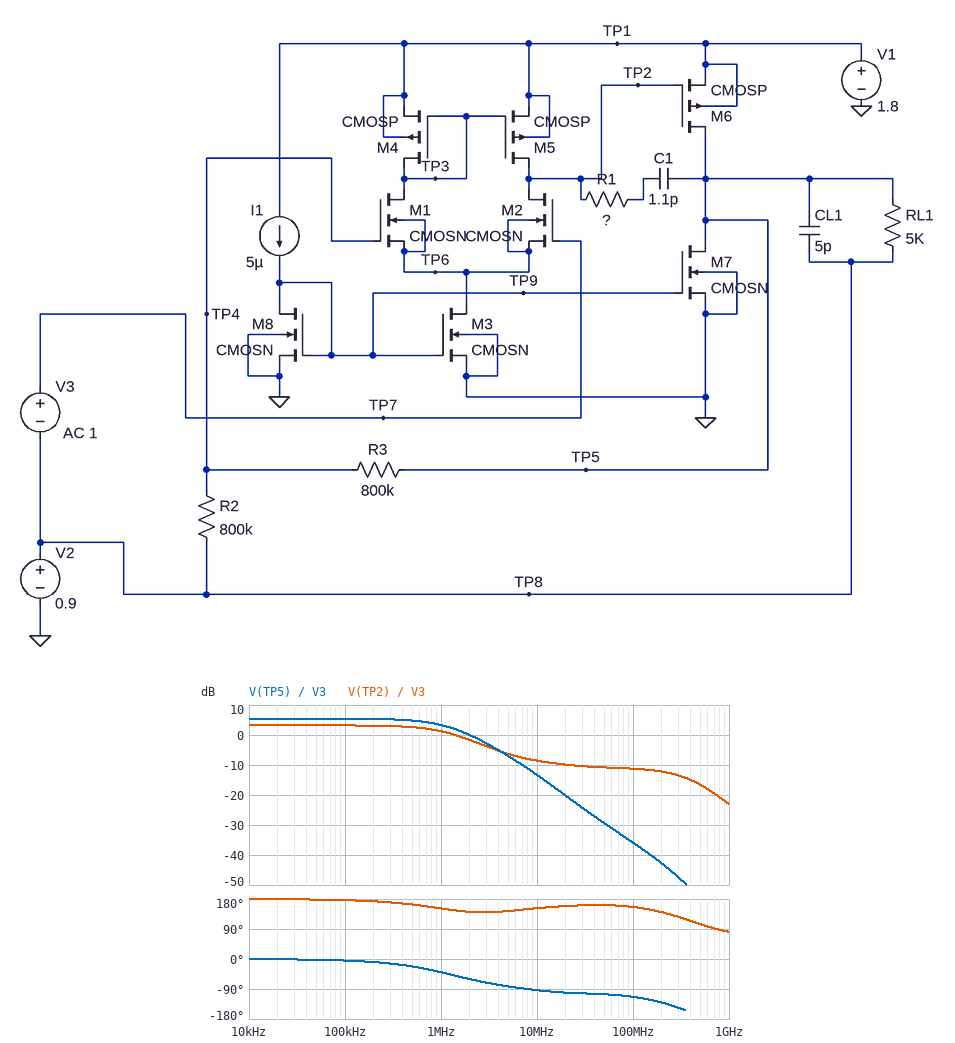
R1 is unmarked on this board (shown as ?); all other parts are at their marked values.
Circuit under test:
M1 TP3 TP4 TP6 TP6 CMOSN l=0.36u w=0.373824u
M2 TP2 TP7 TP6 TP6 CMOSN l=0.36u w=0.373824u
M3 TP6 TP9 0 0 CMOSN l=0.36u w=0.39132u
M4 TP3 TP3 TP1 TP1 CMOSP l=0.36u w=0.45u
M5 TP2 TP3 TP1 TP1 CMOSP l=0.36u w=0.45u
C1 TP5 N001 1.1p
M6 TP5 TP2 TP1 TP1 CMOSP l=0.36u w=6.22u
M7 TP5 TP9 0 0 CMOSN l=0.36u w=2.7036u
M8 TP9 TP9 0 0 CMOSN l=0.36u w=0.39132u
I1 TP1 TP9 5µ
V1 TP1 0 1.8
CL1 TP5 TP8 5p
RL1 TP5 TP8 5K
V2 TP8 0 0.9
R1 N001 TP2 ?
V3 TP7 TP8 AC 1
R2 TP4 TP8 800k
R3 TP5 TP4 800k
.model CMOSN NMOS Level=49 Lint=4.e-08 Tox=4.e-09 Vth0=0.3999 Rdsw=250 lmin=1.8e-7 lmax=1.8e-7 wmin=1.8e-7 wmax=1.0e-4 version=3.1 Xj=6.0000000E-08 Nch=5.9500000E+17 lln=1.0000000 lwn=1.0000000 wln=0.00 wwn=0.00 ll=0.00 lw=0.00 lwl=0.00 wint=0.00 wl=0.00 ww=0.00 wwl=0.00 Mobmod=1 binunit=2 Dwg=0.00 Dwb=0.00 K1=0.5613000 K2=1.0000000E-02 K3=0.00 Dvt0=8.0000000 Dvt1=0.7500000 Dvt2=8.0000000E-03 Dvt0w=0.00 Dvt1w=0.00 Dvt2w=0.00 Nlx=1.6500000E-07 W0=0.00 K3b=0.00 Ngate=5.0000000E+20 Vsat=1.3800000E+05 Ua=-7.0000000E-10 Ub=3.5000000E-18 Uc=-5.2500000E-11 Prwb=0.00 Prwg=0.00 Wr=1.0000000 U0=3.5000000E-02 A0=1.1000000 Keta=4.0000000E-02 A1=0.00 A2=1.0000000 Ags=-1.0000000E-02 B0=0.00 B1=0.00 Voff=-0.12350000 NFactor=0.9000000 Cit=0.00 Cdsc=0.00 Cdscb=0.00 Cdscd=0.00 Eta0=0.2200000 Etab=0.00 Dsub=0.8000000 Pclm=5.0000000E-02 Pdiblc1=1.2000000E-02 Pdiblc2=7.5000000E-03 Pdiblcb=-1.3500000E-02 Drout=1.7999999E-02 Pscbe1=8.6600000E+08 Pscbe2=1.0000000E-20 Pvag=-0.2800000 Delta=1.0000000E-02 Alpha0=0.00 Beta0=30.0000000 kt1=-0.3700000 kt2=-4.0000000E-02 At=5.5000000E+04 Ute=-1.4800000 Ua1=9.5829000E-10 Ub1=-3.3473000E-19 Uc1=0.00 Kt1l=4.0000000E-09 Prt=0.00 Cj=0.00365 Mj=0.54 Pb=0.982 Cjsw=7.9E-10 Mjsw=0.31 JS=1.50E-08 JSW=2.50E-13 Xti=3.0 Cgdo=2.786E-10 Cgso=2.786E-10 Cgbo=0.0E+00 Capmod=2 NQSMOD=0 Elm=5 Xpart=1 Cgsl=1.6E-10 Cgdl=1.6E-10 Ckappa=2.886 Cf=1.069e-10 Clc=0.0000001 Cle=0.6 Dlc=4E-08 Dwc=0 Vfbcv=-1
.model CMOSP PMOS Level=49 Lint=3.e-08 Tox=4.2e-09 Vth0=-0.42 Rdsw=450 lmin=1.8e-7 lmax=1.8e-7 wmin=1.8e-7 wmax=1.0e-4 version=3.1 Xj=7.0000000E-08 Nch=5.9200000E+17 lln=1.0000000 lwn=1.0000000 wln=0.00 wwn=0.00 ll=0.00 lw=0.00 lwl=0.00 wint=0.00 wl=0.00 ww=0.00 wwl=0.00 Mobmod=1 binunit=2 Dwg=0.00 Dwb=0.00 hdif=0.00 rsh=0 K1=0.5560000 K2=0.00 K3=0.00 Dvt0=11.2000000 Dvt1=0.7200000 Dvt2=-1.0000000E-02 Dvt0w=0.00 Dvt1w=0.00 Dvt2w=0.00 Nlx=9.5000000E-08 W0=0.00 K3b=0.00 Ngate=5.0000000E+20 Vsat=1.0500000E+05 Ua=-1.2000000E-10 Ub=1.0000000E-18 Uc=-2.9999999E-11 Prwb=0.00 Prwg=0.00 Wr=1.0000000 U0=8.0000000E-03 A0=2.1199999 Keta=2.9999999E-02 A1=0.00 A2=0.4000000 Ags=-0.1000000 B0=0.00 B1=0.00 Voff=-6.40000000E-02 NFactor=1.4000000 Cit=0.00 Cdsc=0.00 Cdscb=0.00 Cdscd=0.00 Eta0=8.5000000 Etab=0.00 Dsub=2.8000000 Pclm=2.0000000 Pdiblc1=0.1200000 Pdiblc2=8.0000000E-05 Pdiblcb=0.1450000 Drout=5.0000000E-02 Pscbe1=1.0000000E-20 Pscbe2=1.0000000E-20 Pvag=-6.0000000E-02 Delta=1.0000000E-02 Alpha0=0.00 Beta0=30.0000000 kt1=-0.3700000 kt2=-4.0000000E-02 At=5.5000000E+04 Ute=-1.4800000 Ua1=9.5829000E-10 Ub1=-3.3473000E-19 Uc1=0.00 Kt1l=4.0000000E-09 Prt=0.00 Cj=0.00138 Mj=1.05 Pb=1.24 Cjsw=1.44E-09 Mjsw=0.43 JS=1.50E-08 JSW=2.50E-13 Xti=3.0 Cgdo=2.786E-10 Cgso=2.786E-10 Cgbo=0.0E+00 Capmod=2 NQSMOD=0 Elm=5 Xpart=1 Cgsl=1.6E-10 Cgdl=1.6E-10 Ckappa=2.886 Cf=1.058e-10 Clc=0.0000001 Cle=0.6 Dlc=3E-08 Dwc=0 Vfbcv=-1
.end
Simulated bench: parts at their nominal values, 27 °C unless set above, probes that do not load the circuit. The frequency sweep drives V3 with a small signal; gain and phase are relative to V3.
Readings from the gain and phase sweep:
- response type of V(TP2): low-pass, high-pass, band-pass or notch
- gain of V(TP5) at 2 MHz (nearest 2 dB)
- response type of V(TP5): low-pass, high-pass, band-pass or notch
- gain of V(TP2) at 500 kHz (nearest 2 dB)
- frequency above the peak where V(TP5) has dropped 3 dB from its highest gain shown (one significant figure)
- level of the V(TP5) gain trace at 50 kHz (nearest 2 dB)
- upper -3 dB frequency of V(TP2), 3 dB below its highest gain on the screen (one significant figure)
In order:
low-pass
0 dB
low-pass
2 dB
1 MHz
6 dB
1 MHz
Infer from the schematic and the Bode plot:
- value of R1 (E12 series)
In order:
10 kΩ
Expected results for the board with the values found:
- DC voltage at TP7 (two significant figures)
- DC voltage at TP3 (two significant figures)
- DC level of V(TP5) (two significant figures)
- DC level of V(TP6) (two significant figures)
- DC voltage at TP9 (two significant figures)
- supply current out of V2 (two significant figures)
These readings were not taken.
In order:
900 mV
1.1 V
900 mV
290 mV
680 mV
160 nA
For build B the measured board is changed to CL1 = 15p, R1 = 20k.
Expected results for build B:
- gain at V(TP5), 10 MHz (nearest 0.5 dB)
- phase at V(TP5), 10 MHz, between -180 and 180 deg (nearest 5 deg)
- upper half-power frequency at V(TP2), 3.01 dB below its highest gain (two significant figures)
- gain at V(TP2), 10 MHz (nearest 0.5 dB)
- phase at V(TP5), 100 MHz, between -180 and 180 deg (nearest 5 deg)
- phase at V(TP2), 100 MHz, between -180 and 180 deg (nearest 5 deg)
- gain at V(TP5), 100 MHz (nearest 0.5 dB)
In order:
-15.5 dB
-100 deg
2.3 MHz
-3.5 dB
-120 deg
150 deg
-37.5 dB
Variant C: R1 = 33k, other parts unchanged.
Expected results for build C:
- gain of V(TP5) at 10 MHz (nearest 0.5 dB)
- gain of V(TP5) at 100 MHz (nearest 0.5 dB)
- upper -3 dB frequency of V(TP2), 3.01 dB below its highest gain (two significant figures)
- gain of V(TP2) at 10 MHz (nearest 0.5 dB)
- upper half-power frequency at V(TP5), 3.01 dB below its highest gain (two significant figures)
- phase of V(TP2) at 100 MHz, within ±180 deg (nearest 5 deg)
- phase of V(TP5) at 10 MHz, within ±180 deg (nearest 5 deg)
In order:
-8.0 dB
-23.5 dB
1.2 MHz
-4.0 dB
1.1 MHz
150 deg
-50 deg
